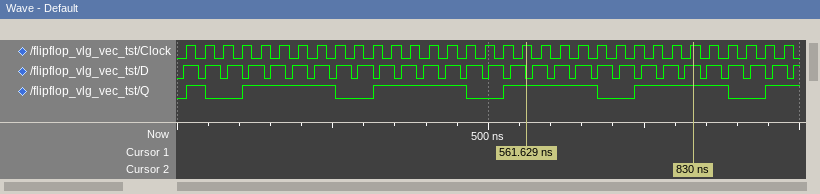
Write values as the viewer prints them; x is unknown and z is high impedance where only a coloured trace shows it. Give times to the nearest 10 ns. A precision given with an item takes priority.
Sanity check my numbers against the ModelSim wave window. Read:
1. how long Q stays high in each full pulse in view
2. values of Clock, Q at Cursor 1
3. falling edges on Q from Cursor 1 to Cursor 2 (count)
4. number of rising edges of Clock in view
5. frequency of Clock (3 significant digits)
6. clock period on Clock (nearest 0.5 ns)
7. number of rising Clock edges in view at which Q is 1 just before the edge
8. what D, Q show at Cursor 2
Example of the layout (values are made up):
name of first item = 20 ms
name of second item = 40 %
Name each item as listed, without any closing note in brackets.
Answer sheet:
how long Q stays high in each full pulse in view = 30 ns, 150 ns, 150 ns, 150 ns, 150 ns
values of Clock, Q at Cursor 1 = Clock=1, Q=1
falling edges on Q from Cursor 1 to Cursor 2 = 1
number of rising edges of Clock in view = 33
frequency of Clock = 33.3 MHz
clock period on Clock = 30 ns
number of rising Clock edges in view at which Q is 1 just before the edge = 22
what D, Q show at Cursor 2 = D=1, Q=1
